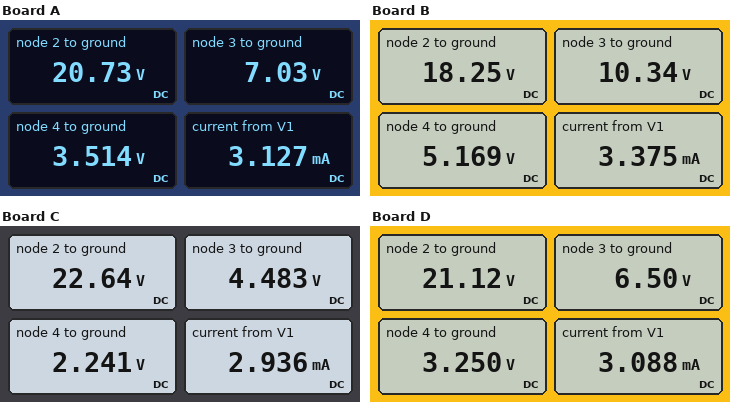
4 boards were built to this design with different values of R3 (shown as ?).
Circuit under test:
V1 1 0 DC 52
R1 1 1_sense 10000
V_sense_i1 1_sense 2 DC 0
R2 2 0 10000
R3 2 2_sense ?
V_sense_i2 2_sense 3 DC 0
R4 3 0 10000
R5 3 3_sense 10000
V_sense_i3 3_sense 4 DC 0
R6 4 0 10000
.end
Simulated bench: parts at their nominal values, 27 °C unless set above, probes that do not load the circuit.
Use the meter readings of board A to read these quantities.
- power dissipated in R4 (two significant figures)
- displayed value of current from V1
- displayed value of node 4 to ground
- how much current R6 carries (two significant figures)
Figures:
4.9 mW
3.127 mA
3.514 V
350 µA
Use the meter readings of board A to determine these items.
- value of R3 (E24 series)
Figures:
13 kΩ
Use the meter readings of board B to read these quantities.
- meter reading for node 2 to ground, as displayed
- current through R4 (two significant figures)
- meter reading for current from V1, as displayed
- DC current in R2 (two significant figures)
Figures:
18.25 V
1.0 mA
3.375 mA
1.8 mA
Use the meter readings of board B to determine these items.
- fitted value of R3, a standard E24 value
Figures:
5.1 kΩ
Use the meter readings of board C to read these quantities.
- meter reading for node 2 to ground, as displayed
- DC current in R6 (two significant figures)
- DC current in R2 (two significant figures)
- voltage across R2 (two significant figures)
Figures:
22.64 V
220 µA
2.3 mA
23 V
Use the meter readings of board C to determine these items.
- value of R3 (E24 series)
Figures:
27 kΩ
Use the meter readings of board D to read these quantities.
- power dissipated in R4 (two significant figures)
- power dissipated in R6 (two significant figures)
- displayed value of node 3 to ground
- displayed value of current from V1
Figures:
4.2 mW
1.1 mW
6.50 V
3.088 mA
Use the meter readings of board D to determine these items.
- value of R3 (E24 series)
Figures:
15 kΩ
